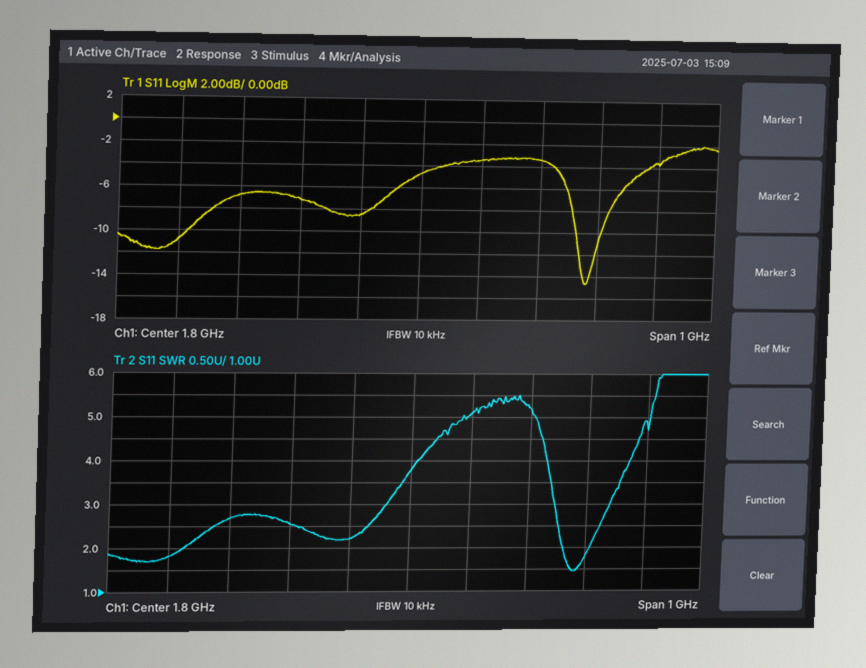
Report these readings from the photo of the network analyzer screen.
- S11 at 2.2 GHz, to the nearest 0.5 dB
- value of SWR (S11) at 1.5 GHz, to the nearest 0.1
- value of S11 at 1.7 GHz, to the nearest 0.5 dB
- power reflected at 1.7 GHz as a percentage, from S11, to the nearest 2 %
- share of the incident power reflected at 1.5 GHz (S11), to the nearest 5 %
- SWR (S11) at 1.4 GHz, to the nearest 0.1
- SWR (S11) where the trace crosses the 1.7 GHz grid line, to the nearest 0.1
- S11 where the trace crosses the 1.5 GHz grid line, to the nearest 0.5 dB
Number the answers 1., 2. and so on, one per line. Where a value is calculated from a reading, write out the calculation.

1. -3.5 dB
2. 2.7
3. -8.5 dB
4. 10^(-8.5/10) ≈ 14 %
5. 10^(-7/10) ≈ 20 %
6. 1.8
7. 2.2
8. -7.0 dB
